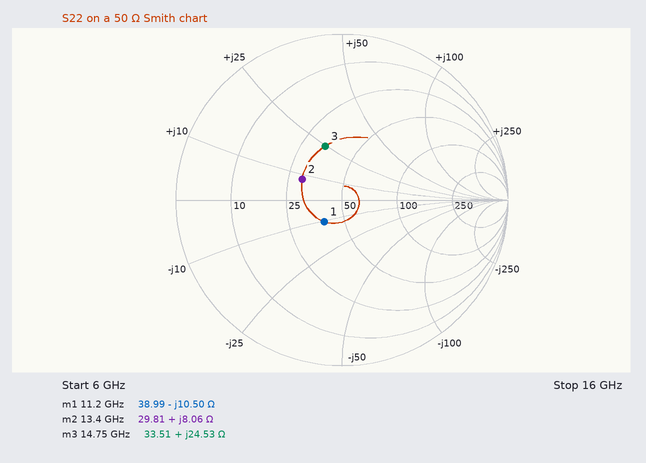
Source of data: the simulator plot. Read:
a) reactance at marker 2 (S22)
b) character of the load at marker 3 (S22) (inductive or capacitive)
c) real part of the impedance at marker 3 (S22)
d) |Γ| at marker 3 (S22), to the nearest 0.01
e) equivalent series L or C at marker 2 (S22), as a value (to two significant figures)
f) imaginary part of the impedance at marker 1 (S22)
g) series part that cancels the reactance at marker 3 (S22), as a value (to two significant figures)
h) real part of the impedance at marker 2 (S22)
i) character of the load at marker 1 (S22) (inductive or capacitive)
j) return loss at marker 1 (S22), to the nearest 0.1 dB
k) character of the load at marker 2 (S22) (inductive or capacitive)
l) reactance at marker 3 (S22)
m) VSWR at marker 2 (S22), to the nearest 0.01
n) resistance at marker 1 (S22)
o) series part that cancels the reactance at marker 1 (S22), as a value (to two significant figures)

+8.06 Ω
inductive
33.51 Ω
0.34
96 pH
-10.50 Ω
440 fF
29.81 Ω
capacitive
15.4 dB
inductive
+24.53 Ω
1.74
38.99 Ω
150 pH
